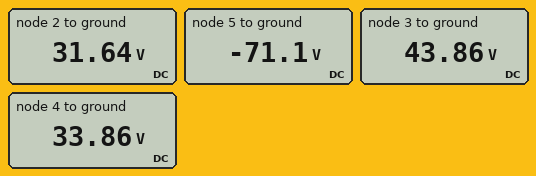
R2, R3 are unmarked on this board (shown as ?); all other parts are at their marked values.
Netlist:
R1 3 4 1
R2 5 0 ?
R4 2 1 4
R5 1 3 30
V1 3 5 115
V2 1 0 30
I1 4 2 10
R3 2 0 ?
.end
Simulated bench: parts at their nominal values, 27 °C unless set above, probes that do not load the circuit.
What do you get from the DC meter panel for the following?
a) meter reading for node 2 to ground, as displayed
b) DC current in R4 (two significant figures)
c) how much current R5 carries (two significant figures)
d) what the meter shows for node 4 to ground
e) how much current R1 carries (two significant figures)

31.64 V
410 mA
460 mA
33.86 V
10 A
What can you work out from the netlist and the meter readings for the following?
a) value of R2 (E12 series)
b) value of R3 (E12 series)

6.8 Ω
3.3 Ω
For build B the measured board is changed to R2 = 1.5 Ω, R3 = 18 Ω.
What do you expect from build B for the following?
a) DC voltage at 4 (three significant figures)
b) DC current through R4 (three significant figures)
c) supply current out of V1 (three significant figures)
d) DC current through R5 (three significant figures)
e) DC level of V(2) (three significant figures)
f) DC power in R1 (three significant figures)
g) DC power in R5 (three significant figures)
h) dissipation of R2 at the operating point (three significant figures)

86.7 V
6.82 A
12.2 A
2.22 A
57.3 V
100 W
148 W
224 W
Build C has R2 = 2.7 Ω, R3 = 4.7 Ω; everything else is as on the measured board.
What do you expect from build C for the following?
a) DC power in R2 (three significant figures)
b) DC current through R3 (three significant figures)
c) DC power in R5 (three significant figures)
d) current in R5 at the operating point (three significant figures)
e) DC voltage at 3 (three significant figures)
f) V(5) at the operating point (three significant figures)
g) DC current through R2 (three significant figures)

374 W
8.05 A
94.4 W
1.77 A
83.2 V
-31.8 V
11.8 A
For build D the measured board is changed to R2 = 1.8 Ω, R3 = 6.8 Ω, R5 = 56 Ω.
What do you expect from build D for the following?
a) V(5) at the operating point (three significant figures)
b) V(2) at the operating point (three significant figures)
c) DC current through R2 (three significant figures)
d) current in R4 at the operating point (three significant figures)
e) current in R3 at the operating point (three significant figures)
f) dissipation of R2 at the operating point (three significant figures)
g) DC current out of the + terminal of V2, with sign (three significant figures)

-20.1 V
44.1 V
11.2 A
3.52 A
6.48 A
224 W
-4.68 A
